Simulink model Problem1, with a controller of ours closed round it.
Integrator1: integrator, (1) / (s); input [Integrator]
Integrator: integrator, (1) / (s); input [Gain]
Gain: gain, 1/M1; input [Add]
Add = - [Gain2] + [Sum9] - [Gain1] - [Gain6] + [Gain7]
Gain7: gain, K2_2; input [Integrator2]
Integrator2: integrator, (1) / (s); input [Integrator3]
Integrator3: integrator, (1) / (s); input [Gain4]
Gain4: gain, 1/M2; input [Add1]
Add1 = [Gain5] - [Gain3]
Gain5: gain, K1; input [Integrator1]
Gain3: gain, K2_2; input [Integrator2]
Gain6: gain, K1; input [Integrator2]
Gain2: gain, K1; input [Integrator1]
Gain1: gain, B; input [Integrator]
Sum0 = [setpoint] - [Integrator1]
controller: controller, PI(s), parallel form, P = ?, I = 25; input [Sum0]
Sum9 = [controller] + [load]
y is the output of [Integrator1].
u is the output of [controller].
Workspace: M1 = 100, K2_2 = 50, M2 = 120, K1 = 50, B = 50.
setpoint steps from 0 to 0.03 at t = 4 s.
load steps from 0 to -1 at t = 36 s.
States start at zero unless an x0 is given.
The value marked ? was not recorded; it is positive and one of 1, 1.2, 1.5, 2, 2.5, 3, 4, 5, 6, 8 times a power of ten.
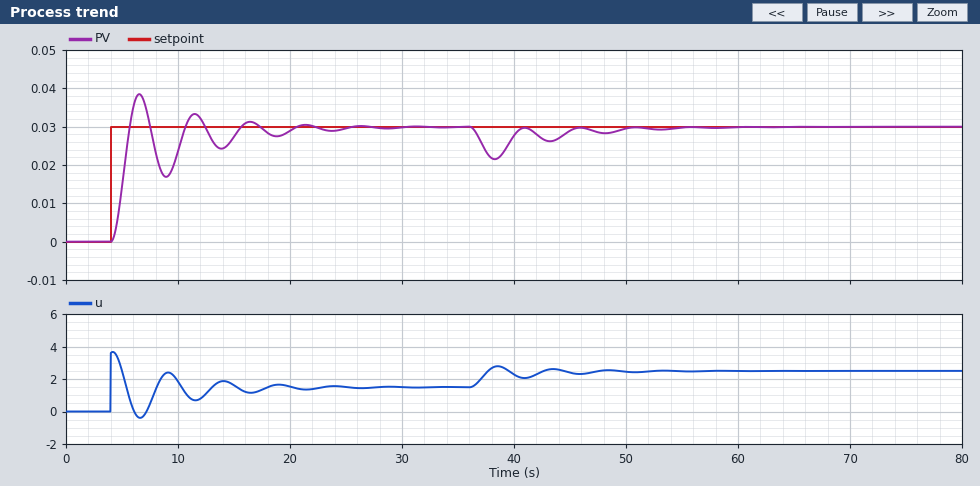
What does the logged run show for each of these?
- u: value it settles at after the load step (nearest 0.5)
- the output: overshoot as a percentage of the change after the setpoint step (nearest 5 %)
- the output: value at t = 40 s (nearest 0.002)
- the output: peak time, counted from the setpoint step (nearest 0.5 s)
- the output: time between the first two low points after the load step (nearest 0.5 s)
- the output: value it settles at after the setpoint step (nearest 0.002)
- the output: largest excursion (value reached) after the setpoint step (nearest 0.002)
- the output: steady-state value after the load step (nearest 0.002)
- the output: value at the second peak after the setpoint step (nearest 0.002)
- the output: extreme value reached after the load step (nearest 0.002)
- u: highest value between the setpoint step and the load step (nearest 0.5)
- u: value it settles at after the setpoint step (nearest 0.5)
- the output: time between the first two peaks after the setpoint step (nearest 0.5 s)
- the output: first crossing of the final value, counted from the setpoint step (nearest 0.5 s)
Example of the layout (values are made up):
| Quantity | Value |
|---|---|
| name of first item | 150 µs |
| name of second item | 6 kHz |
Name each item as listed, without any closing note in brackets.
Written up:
| Quantity | Value |
|---|---|
| u: value it settles at after the load step | 2.5 |
| the output: overshoot as a percentage of the change after the setpoint step | 30 % |
| the output: value at t = 40 s | 0.028 |
| the output: peak time, counted from the setpoint step | 2.5 s |
| the output: time between the first two low points after the load step | 5.0 s |
| the output: value it settles at after the setpoint step | 0.030 |
| the output: largest excursion (value reached) after the setpoint step | 0.038 |
| the output: steady-state value after the load step | 0.030 |
| the output: value at the second peak after the setpoint step | 0.034 |
| the output: extreme value reached after the load step | 0.022 |
| u: highest value between the setpoint step and the load step | 3.5 |
| u: value it settles at after the setpoint step | 1.5 |
| the output: time between the first two peaks after the setpoint step | 5.0 s |
| the output: first crossing of the final value, counted from the setpoint step | 1.5 s |
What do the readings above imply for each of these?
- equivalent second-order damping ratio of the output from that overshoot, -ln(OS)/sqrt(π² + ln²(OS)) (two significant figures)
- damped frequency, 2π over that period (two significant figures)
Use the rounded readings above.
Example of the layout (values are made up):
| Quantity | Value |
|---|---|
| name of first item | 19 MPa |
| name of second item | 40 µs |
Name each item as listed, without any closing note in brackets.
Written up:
| Quantity | Value |
|---|---|
| equivalent second-order damping ratio of the output from that overshoot, -ln(OS)/sqrt(π² + ln²(OS)) | 0.36 |
| damped frequency, 2π over that period | 1.3 rad/s |
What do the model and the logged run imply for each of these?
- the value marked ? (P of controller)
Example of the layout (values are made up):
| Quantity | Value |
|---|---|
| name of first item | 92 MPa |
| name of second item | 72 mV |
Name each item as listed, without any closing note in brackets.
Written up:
| Quantity | Value |
|---|---|
| the value marked ? | 120 |
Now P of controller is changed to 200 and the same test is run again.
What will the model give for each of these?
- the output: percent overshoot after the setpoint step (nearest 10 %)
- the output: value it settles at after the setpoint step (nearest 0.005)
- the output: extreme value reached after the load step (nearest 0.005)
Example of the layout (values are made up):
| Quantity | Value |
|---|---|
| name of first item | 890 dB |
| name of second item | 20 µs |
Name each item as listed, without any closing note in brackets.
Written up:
| Quantity | Value |
|---|---|
| the output: percent overshoot after the setpoint step | 40 % |
| the output: value it settles at after the setpoint step | 0.030 |
| the output: extreme value reached after the load step | 0.025 |
